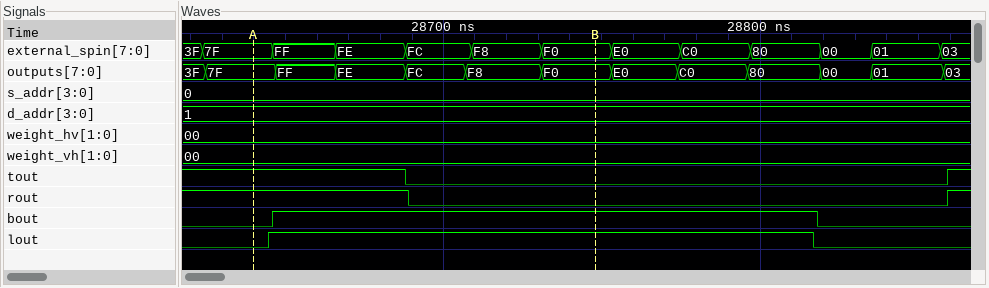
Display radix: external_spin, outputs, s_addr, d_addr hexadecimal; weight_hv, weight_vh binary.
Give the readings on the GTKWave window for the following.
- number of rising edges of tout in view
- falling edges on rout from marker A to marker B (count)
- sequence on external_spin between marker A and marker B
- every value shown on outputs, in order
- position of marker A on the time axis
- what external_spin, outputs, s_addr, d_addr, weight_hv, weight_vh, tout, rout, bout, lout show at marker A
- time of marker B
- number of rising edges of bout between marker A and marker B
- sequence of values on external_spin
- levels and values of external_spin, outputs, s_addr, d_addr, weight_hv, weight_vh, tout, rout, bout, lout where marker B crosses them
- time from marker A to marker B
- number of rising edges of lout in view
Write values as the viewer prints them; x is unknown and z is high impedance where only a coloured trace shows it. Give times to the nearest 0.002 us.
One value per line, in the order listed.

1
1
7F, FF, FE, FC, F8, F0
3F, 7F, FF, FE, FC, F8, F0, E0, C0, 80, 00, 01, 03
28.64 us
external_spin=7F, outputs=7F, s_addr=0, d_addr=1, weight_hv=00, weight_vh=00, tout=1, rout=1, bout=0, lout=0
28.748 us
1
3F, 7F, FF, FE, FC, F8, F0, E0, C0, 80, 00, 01, 03
external_spin=F0, outputs=F0, s_addr=0, d_addr=1, weight_hv=00, weight_vh=00, tout=0, rout=0, bout=1, lout=1
0.108 us
1
